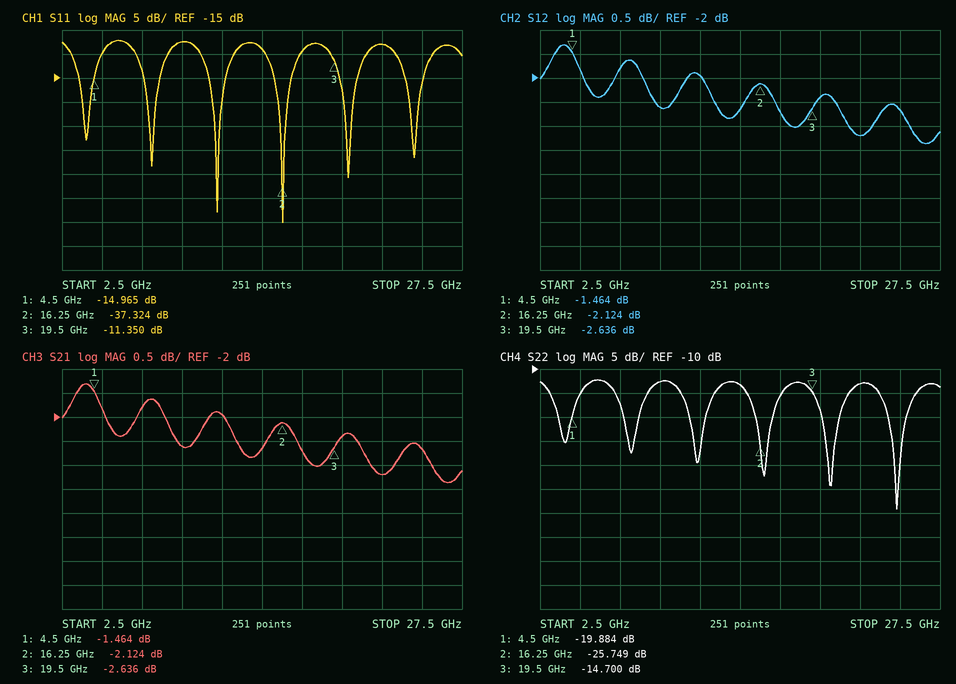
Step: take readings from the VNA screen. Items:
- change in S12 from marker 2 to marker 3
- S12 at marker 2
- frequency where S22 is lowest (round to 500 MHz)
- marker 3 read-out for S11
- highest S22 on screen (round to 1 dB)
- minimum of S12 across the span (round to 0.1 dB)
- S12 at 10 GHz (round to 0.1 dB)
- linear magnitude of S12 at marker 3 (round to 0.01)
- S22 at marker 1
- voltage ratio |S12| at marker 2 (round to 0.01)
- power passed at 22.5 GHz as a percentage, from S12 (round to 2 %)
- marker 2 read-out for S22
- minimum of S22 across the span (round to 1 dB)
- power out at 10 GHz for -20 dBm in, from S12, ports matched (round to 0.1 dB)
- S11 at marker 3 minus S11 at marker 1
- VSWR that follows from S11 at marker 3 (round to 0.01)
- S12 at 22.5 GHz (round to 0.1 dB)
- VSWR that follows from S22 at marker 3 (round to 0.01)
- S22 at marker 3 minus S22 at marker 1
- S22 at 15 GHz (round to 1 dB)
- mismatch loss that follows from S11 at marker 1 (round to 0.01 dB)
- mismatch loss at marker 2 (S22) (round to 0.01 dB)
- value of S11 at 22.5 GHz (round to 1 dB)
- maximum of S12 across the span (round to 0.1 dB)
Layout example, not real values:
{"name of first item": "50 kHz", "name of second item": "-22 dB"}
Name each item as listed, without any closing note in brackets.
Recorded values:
{"change in S12 from marker 2 to marker 3": "-0.512 dB", "S12 at marker 2": "-2.124 dB", "frequency where S22 is lowest": "25.0 GHz", "marker 3 read-out for S11": "-11.350 dB", "highest S22 on screen": "-12 dB", "minimum of S12 across the span": "-3.4 dB", "S12 at 10 GHz": "-2.6 dB", "linear magnitude of S12 at marker 3": "0.74", "S22 at marker 1": "-19.884 dB", "voltage ratio |S12| at marker 2": "0.78", "power passed at 22.5 GHz as a percentage, from S12": "48 %", "marker 2 read-out for S22": "-25.749 dB", "minimum of S22 across the span": "-39 dB", "power out at 10 GHz for -20 dBm in, from S12, ports matched": "-22.6 dBm", "S11 at marker 3 minus S11 at marker 1": "3.615 dB", "VSWR that follows from S11 at marker 3": "1.74", "S12 at 22.5 GHz": "-3.2 dB", "VSWR that follows from S22 at marker 3": "1.45", "S22 at marker 3 minus S22 at marker 1": "5.184 dB", "S22 at 15 GHz": "-13 dB", "mismatch loss that follows from S11 at marker 1": "0.14 dB", "mismatch loss at marker 2 (S22)": "0.01 dB", "value of S11 at 22.5 GHz": "-8 dB", "maximum of S12 across the span": "-1.3 dB"}
